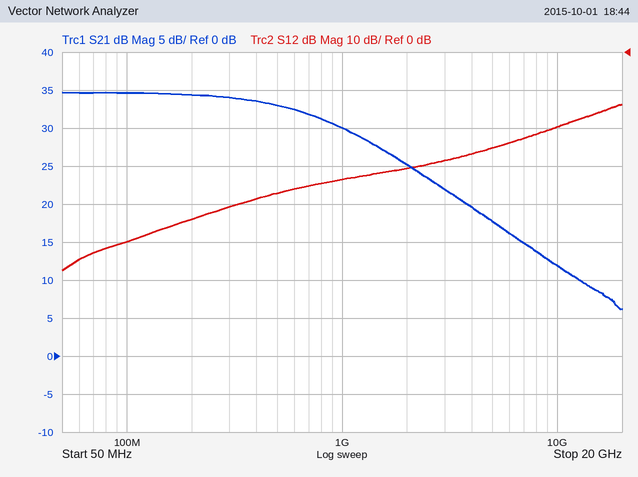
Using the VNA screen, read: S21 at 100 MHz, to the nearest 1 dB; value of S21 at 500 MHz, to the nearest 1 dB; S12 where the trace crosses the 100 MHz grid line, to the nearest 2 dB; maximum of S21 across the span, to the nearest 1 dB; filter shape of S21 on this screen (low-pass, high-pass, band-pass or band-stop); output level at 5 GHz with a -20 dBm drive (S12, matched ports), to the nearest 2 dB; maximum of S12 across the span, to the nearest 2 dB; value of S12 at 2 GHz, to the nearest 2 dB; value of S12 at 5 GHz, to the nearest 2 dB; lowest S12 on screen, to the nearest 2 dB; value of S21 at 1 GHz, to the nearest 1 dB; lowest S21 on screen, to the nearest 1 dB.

35 dB
33 dB
-50 dB
35 dB
low-pass
-46 dBm
-14 dB
-30 dB
-26 dB
-58 dB
30 dB
6 dB
